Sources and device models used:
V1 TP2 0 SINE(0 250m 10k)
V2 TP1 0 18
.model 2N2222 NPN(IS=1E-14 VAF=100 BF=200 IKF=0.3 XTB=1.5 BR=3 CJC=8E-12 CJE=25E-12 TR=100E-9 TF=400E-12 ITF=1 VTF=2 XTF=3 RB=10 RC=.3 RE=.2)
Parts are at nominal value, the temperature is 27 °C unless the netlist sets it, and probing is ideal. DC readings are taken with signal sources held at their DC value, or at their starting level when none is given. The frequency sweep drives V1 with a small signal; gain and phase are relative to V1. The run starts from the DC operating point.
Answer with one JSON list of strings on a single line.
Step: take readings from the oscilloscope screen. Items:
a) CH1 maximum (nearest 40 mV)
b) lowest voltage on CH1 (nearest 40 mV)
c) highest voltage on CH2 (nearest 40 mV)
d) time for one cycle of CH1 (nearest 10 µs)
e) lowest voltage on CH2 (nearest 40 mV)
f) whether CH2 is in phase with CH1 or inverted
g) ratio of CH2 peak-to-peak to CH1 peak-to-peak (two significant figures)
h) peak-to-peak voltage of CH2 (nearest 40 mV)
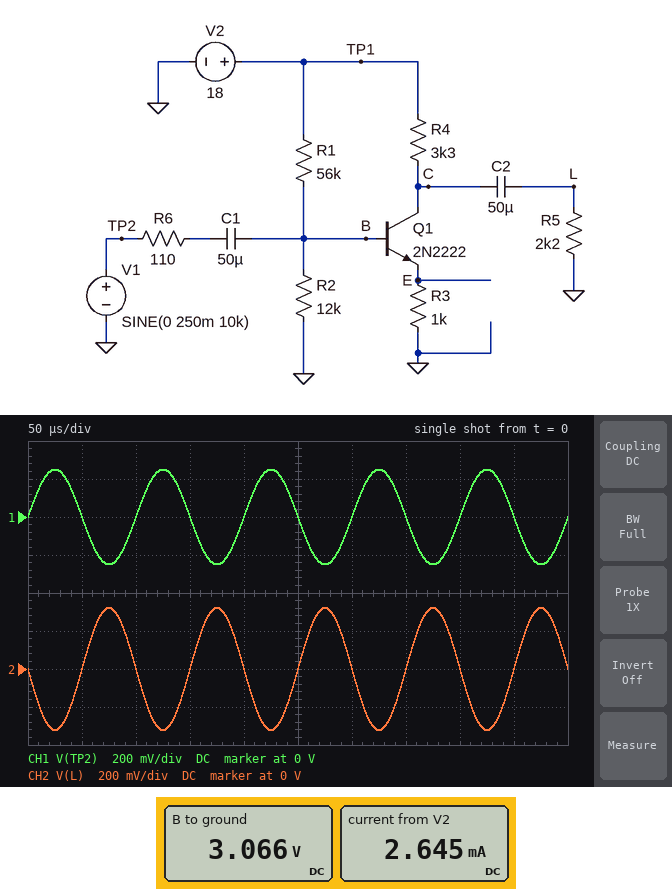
["240 mV", "-240 mV", "320 mV", "100 µs", "-320 mV", "inverted", "1.3", "640 mV"]
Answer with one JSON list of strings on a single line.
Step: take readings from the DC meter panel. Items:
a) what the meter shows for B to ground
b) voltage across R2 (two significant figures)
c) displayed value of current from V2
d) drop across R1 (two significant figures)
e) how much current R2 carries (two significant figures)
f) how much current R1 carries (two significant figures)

["3.066 V", "3.1 V", "2.645 mA", "15 V", "260 µA", "270 µA"]
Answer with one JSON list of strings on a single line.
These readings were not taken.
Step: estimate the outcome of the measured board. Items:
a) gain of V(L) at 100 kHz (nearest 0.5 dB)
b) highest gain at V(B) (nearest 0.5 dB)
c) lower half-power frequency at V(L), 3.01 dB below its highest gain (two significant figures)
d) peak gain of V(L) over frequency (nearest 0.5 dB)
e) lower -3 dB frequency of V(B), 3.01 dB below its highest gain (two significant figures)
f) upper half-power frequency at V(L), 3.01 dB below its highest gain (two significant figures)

["2.0 dB", "0 dB", "720 mHz", "2.0 dB", "330 mHz", "170 MHz"]
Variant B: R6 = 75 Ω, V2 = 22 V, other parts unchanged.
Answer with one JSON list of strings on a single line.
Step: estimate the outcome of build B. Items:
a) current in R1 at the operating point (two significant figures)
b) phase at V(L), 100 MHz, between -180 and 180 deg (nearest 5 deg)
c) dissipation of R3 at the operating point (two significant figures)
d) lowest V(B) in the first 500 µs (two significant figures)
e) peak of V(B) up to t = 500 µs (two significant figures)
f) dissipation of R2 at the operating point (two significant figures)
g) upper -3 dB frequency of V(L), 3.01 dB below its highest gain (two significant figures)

["330 µA", "35 deg", "9.4 mW", "3.5 V", "4.0 V", "1.2 mW", "320 MHz"]
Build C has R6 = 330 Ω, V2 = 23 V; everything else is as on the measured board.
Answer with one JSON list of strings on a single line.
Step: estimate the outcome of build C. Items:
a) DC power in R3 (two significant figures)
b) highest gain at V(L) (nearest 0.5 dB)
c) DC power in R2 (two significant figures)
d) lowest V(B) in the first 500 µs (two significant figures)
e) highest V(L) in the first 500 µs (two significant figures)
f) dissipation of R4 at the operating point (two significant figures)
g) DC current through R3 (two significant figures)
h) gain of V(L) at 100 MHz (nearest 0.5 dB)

["10 mW", "2.0 dB", "1.3 mW", "3.7 V", "310 mV", "34 mW", "3.2 mA", "-3.0 dB"]
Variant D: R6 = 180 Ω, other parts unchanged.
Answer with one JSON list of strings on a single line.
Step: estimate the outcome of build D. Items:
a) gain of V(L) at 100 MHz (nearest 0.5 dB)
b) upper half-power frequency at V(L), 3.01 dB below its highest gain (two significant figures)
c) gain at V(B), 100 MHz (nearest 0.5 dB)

["-1.5 dB", "66 MHz", "-2.5 dB"]
